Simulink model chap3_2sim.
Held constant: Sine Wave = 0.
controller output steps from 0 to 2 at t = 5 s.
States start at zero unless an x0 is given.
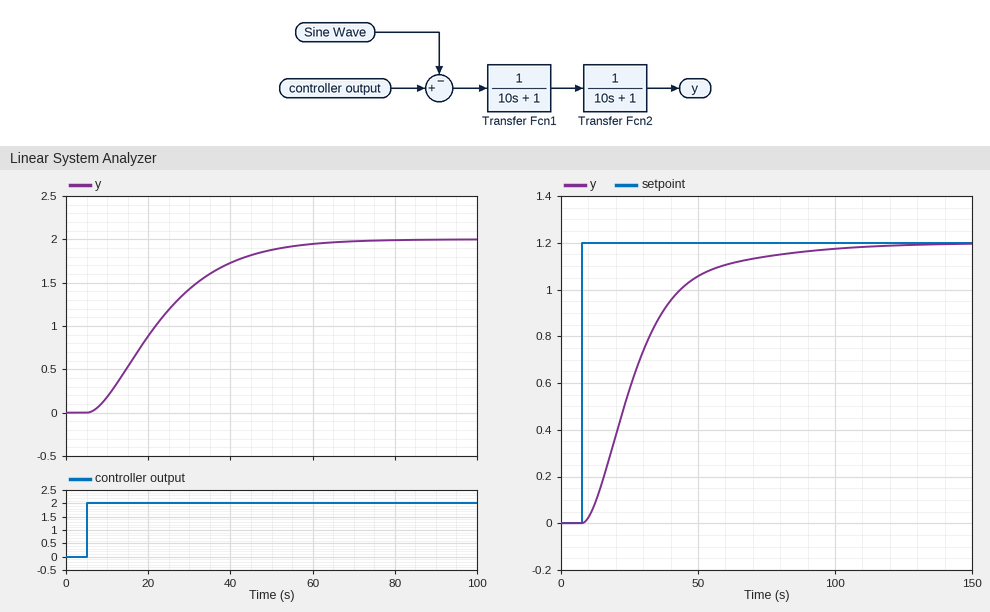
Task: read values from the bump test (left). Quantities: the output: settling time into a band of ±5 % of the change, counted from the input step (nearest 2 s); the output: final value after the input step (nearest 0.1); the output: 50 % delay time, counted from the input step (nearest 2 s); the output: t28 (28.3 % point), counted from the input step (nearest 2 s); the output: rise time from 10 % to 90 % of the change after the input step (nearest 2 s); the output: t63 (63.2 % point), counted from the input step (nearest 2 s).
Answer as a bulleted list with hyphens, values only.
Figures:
- 48 s
- 2.0
- 16 s
- 10 s
- 34 s
- 22 s
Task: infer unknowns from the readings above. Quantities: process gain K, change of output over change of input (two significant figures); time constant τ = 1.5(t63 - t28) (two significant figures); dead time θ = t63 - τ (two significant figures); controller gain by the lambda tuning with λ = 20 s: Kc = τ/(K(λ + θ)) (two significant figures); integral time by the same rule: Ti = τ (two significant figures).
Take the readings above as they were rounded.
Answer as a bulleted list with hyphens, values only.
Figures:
- 1.0
- 18 s
- 4.0 s
- 0.75
- 18 s
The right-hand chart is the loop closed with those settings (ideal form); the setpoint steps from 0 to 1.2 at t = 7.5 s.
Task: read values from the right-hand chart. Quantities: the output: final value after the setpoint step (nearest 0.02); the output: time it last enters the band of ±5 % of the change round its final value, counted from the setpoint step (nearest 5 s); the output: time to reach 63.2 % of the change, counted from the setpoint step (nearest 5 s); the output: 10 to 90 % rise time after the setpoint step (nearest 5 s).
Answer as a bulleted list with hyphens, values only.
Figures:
- 1.20
- 65 s
- 25 s
- 40 s
